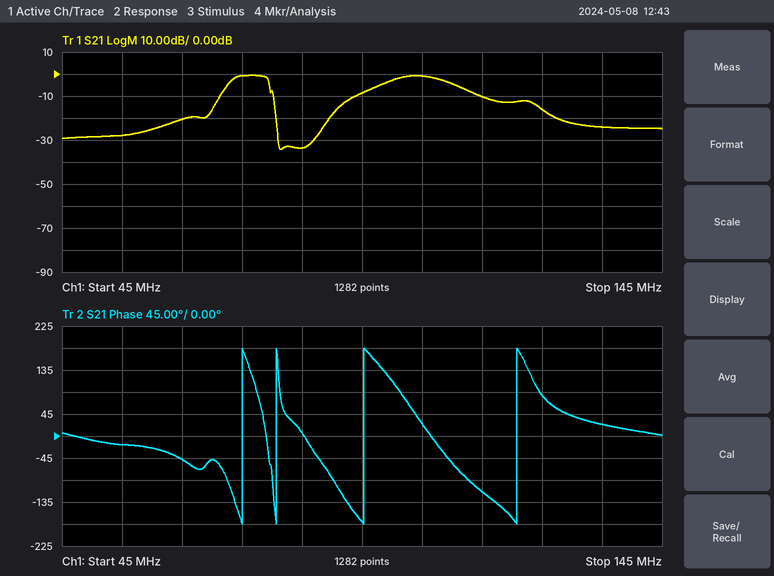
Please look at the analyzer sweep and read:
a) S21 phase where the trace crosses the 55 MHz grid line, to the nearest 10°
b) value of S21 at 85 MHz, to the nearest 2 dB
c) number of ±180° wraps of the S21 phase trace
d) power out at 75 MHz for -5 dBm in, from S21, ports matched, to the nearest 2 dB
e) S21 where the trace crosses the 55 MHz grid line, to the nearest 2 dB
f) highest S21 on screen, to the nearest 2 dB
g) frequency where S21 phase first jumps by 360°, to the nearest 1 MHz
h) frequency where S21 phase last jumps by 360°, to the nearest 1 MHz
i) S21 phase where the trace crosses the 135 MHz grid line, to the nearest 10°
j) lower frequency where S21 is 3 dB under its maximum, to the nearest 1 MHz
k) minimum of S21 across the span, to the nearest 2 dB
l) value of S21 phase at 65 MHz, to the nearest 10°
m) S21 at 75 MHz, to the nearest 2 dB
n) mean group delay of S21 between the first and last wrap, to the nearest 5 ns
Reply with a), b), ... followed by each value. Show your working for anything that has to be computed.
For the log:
a) -20°
b) -34 dB
c) 4
d) -5 dBm + (0 dB) = -6 dBm
e) -28 dB
f) 0 dB
g) 75 MHz
h) 121 MHz
i) 20°
j) 73 MHz
k) -34 dB
l) -50°
m) 0 dB
n) 3 cycles / (121 MHz − 75 MHz) ≈ 65 ns
